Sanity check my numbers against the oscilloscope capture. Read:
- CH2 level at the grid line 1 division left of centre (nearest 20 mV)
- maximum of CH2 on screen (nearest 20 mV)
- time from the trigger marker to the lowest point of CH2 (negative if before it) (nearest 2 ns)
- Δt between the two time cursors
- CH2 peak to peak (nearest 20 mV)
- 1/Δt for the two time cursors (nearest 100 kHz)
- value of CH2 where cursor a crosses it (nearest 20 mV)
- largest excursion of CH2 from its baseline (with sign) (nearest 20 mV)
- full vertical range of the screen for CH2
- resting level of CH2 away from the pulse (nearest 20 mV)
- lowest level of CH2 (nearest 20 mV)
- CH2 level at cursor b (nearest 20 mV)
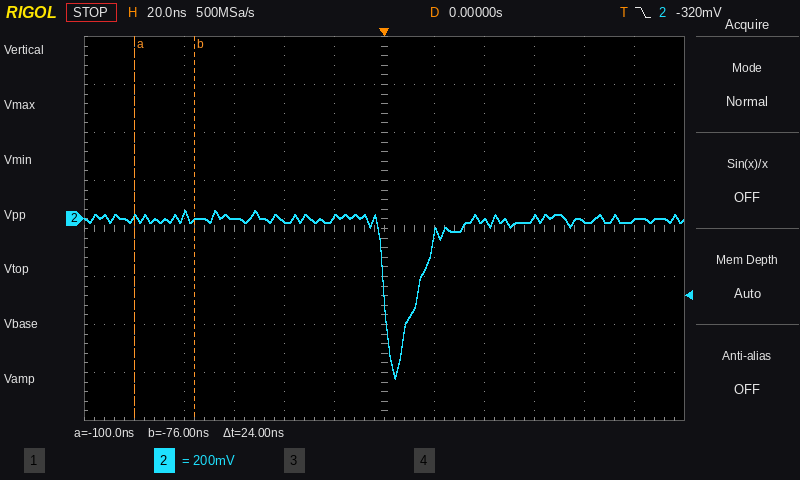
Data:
0 mV
40 mV
+4 ns
24 ns
700 mV
41.7 MHz
0 mV
-660 mV
1.6 V
0 mV
-660 mV
0 mV
